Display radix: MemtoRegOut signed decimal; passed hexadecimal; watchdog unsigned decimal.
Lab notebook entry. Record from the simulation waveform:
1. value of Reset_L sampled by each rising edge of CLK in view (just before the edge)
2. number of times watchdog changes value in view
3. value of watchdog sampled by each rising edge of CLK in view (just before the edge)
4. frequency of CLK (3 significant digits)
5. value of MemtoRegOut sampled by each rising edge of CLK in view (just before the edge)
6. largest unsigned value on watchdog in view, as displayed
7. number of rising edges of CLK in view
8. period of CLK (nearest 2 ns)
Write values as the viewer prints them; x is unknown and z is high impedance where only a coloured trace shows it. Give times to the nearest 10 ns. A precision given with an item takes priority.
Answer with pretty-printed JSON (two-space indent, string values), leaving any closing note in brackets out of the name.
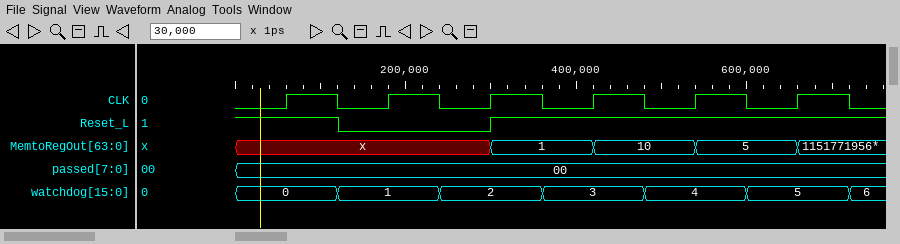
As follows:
{
  "value of Reset_L sampled by each rising edge of CLK in view": "1 0 0 1 1 1",
  "number of times watchdog changes value in view": "6",
  "value of watchdog sampled by each rising edge of CLK in view": "0, 1, 2, 3, 4, 5",
  "frequency of CLK": "8.33 MHz",
  "value of MemtoRegOut sampled by each rising edge of CLK in view": "x, x, x, 1, 10, 5",
  "largest unsigned value on watchdog in view, as displayed": "6",
  "number of rising edges of CLK in view": "6",
  "period of CLK": "120 ns"
}
